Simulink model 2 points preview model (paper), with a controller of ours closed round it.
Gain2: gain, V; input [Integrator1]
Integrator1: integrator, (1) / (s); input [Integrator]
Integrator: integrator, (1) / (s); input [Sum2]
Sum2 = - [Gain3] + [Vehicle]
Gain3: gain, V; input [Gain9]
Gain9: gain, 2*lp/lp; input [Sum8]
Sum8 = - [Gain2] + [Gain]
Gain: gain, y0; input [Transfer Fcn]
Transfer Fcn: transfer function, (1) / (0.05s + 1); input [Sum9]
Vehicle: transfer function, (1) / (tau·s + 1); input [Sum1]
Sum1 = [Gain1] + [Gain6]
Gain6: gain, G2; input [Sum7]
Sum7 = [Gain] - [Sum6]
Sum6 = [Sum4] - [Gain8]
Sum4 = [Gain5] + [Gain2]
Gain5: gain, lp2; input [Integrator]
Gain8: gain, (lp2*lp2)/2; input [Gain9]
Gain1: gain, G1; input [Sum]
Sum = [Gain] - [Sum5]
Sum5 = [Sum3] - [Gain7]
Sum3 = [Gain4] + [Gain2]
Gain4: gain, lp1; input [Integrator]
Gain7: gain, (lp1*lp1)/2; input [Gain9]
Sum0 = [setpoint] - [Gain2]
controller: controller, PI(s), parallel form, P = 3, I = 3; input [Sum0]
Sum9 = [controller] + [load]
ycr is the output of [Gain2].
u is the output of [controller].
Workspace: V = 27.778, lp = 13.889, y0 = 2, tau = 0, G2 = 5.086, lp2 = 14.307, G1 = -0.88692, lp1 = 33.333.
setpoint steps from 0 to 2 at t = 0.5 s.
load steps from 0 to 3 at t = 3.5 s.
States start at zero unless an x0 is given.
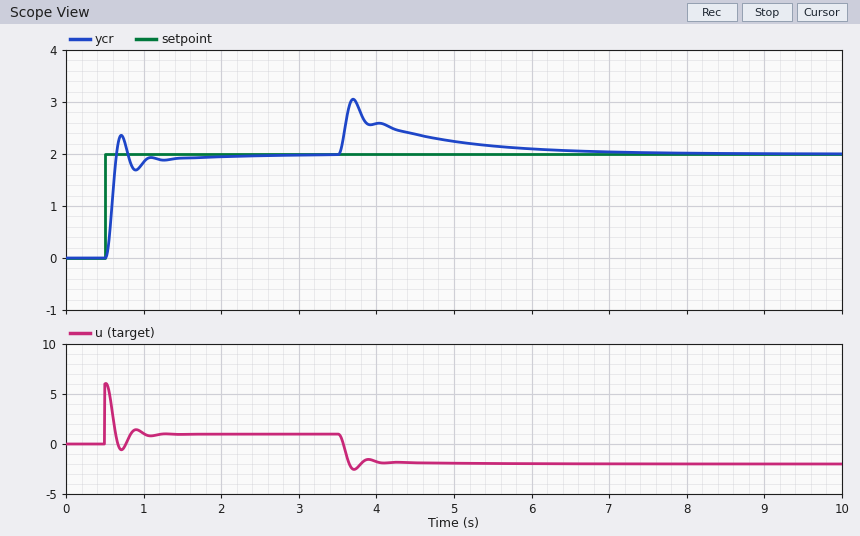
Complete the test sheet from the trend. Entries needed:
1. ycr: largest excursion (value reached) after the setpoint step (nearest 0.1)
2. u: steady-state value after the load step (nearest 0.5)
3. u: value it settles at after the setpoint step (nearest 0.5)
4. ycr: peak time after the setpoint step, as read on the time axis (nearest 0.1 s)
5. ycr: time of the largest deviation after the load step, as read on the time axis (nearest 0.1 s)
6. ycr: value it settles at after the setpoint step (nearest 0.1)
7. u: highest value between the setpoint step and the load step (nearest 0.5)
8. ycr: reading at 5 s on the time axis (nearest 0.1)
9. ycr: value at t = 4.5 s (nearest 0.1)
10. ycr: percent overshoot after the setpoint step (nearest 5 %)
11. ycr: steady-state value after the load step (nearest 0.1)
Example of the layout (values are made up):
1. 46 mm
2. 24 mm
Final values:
1. 2.4
2. -2.0
3. 1.0
4. 0.7 s
5. 3.7 s
6. 2.0
7. 6.0
8. 2.2
9. 2.4
10. 20 %
11. 2.0
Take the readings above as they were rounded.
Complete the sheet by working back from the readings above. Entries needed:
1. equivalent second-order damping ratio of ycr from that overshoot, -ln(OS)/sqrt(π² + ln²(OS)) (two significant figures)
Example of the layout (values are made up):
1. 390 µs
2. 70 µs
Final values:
1. 0.46
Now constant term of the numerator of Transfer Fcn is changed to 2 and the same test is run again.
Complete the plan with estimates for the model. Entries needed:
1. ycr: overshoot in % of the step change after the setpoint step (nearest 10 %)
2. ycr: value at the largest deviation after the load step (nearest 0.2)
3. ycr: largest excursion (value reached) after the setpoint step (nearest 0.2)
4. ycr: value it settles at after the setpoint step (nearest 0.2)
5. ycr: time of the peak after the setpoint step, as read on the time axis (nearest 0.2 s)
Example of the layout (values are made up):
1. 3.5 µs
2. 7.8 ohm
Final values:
1. 50 %
2. 3.4
3. 3.0
4. 2.0
5. 0.6 s
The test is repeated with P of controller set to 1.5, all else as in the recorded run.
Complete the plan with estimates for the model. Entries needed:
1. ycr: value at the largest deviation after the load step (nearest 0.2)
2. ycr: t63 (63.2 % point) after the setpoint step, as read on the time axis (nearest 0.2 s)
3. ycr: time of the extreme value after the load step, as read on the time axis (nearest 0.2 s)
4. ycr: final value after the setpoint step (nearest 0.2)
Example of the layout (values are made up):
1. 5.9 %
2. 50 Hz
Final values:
1. 3.6
2. 0.6 s
3. 3.8 s
4. 2.0
